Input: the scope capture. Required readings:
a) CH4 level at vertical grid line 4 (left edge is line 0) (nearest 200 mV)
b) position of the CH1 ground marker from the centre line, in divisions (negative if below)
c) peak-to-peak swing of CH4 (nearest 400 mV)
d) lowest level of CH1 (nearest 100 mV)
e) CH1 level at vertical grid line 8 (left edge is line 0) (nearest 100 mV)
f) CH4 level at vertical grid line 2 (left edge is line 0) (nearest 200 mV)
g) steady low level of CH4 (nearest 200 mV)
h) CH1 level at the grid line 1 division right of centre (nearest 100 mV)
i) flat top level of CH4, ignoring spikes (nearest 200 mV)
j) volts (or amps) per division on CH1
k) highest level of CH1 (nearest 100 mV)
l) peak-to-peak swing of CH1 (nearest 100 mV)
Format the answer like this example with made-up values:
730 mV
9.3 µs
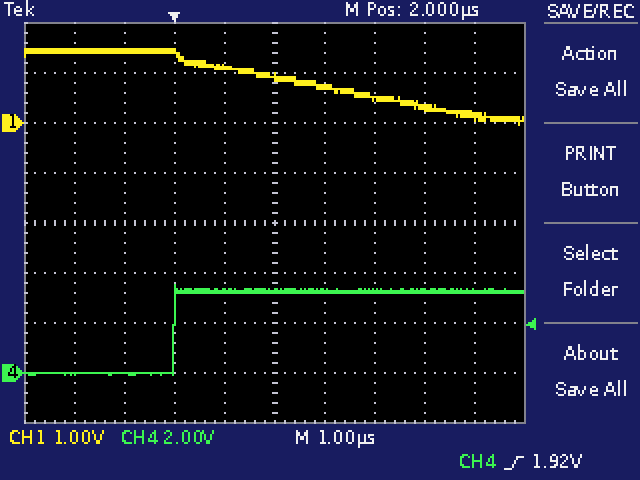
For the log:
3.2 V
+2.0 div
3.6 V
0.0 V
300 mV
0.0 V
0.0 V
700 mV
3.2 V
1 V
1.5 V
1.5 V
